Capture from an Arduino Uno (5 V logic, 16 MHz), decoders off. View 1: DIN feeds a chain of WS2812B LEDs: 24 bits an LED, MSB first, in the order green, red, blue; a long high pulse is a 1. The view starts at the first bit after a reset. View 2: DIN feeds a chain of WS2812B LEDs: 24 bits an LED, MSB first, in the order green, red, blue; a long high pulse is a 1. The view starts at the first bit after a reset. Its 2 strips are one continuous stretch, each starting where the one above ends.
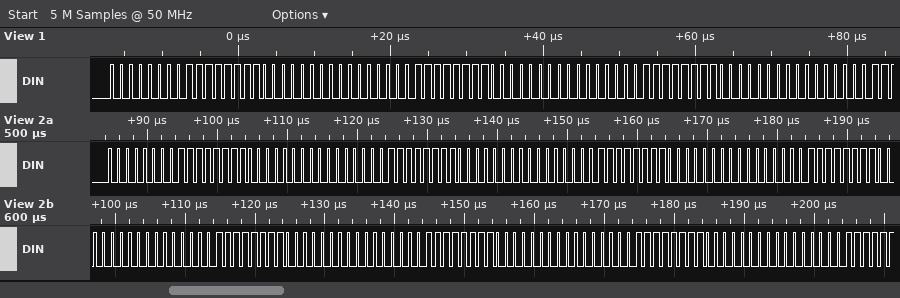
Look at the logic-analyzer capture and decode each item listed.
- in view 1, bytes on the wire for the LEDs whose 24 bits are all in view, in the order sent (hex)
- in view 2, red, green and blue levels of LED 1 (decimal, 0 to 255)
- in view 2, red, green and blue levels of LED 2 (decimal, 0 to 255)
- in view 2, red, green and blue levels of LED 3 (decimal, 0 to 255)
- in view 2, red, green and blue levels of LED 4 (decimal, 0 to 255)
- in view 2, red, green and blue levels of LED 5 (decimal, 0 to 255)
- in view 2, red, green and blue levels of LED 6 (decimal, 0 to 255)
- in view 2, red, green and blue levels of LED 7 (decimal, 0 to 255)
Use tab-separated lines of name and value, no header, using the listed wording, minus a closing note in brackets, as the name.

in view 1, bytes on the wire for the LEDs whose 24 bits are all in view, in the order sent	00 FF 00 00 FF 00 00 FF 00
in view 2, red, green and blue levels of LED 1	255, 0, 0
in view 2, red, green and blue levels of LED 2	255, 0, 0
in view 2, red, green and blue levels of LED 3	255, 0, 0
in view 2, red, green and blue levels of LED 4	255, 0, 0
in view 2, red, green and blue levels of LED 5	255, 0, 0
in view 2, red, green and blue levels of LED 6	255, 0, 0
in view 2, red, green and blue levels of LED 7	255, 0, 0
